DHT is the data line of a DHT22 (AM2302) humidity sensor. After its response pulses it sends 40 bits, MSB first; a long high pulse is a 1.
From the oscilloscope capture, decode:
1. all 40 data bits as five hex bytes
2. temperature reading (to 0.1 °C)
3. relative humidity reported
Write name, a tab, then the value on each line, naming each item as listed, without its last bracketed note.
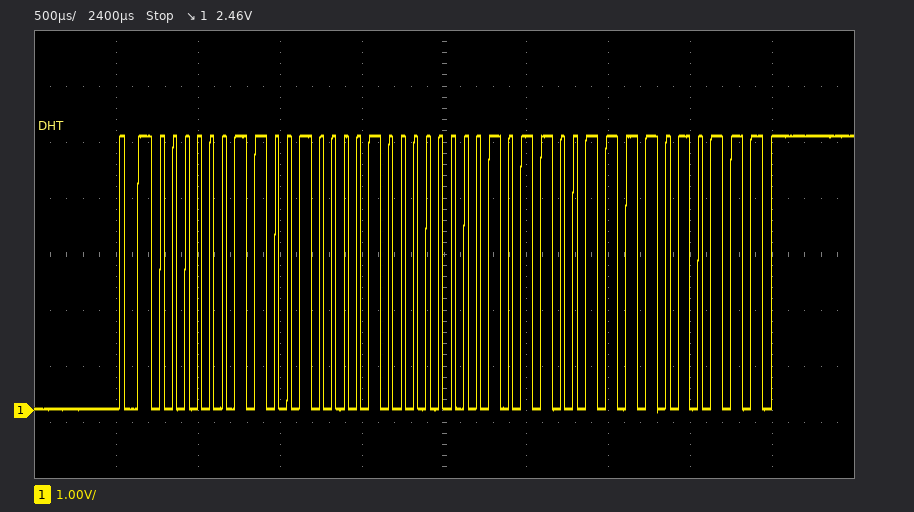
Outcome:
all 40 data bits as five hex bytes	03 21 00 B3 D7
temperature reading	17.9 °C
relative humidity reported	80.1 %
